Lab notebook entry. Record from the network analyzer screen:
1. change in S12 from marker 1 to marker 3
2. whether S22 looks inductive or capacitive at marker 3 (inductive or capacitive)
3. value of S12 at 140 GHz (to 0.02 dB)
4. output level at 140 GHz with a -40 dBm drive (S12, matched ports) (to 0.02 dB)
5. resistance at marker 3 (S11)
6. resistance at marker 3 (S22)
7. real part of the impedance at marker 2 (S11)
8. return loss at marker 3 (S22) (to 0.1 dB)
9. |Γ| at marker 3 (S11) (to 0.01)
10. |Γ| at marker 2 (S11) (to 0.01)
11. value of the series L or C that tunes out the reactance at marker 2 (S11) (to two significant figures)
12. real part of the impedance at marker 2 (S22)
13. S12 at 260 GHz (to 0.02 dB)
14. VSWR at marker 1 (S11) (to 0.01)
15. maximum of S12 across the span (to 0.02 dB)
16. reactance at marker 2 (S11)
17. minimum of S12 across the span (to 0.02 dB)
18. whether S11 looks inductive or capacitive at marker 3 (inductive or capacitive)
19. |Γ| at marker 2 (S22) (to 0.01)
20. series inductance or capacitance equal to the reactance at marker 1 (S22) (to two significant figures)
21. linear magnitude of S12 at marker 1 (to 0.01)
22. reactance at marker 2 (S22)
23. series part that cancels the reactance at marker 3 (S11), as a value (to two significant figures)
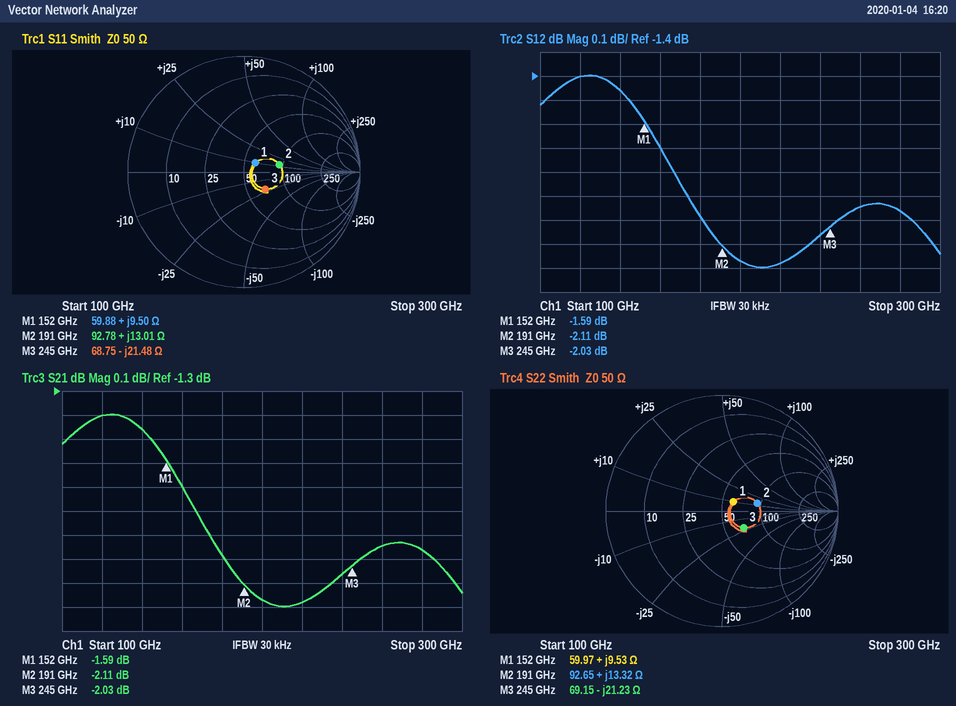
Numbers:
-0.44 dB
capacitive
-1.46 dB
-41.46 dBm
68.75 Ω
69.15 Ω
92.78 Ω
12.5 dB
0.24
0.31
64 fF
92.65 Ω
-1.94 dB
1.28
-1.40 dB
+13.01 Ω
-2.20 dB
capacitive
0.31
10.0 pH
0.83
+13.32 Ω
14 pH
